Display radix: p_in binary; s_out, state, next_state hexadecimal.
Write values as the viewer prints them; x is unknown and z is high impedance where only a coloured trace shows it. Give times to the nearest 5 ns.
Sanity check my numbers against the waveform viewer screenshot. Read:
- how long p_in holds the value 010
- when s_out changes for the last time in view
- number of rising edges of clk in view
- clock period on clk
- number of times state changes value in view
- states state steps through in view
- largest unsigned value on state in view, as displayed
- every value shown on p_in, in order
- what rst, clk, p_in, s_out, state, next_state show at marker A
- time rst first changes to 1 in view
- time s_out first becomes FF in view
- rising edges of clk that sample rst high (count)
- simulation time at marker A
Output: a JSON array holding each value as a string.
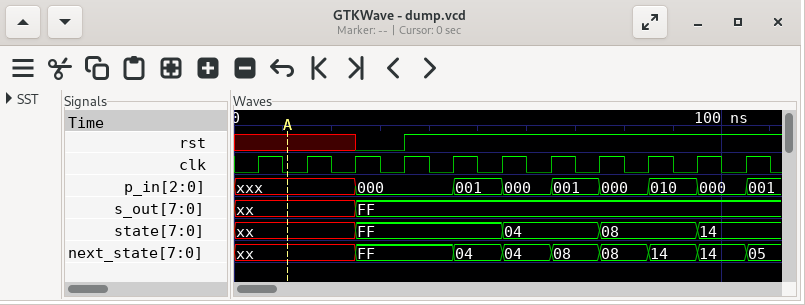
["10 ns", "25 ns", "11", "10 ns", "4", "xx, FF, 04, 08, 14", "FF", "xxx, 000, 001, 000, 001, 000, 010, 000, 001", "rst=x, clk=0, p_in=xxx, s_out=xx, state=xx, next_state=xx", "35 ns", "25 ns", "7", "10 ns"]
